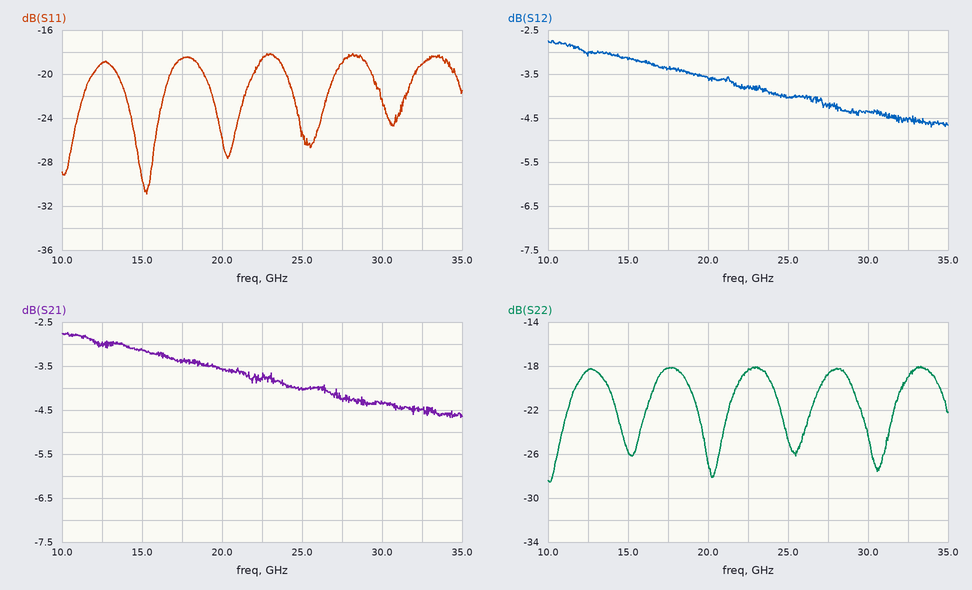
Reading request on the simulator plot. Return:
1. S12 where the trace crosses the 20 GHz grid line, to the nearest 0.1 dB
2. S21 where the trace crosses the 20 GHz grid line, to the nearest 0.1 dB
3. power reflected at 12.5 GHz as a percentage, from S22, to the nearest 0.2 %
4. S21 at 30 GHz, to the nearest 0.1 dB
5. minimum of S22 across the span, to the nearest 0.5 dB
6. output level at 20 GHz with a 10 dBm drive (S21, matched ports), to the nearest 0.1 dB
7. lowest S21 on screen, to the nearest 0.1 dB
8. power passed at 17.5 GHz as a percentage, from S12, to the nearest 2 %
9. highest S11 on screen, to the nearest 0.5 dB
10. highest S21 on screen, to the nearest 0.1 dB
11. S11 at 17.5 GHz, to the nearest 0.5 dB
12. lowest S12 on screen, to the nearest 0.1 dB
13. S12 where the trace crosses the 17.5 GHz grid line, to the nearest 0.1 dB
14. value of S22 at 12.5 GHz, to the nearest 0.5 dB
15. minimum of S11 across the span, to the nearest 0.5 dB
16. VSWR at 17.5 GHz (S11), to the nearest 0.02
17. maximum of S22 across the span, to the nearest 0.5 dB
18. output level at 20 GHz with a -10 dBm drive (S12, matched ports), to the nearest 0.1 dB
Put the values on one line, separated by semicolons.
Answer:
-3.6 dB; -3.6 dB; 1.4 %; -4.3 dB; -28.5 dB; 6.4 dBm; -4.7 dB; 46 %; -18.0 dB; -2.7 dB; -18.5 dB; -4.7 dB; -3.4 dB; -18.5 dB; -31.0 dB; 1.26; -18.0 dB; -13.6 dBm
